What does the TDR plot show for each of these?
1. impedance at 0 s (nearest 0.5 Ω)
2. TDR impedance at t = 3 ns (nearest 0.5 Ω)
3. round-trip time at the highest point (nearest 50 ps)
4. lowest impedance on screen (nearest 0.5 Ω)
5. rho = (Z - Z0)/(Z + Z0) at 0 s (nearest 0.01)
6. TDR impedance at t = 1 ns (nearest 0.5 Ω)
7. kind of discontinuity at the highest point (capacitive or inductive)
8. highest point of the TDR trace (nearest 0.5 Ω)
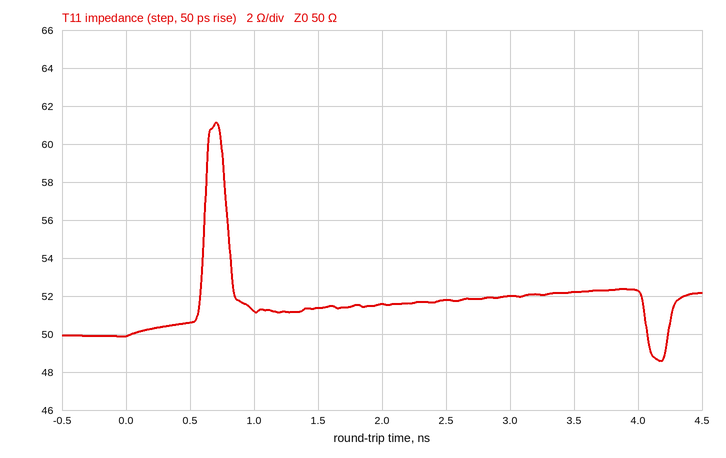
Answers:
50.0 Ω
52.0 Ω
700 ps
48.5 Ω
0.00
51.0 Ω
inductive
61.0 Ω
